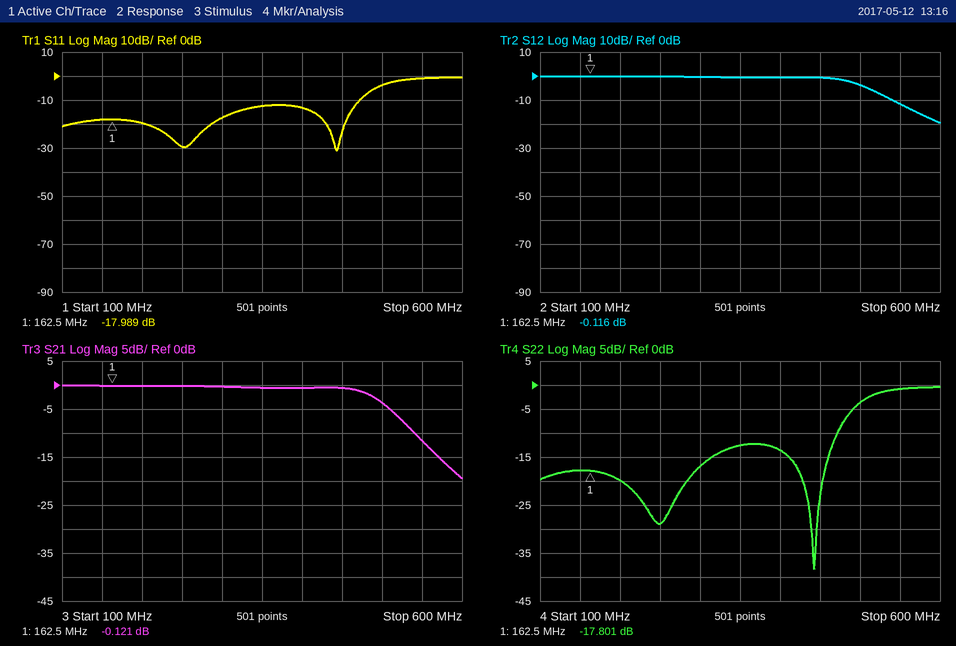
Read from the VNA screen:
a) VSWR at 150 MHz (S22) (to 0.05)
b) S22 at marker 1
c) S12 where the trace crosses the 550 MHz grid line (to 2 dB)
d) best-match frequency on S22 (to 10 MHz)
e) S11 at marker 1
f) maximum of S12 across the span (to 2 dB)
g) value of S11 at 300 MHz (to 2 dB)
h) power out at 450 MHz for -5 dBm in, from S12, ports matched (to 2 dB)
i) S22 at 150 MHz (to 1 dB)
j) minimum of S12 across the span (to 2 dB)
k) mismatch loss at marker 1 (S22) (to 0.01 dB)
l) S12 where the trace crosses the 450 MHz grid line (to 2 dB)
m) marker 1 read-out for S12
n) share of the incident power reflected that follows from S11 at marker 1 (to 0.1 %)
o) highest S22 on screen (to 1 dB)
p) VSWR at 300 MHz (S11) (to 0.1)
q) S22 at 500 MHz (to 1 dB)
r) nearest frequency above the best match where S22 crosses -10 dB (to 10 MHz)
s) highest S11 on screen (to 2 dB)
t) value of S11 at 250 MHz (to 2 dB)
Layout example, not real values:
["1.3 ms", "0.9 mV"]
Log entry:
["1.30", "-17.801 dB", "-12 dB", "440 MHz", "-17.989 dB", "0 dB", "-18 dB", "-6 dBm", "-18 dB", "-20 dB", "0.07 dB", "0 dB", "-0.116 dB", "1.6 %", "0 dB", "1.3", "-4 dB", "470 MHz", "0 dB", "-30 dB"]
